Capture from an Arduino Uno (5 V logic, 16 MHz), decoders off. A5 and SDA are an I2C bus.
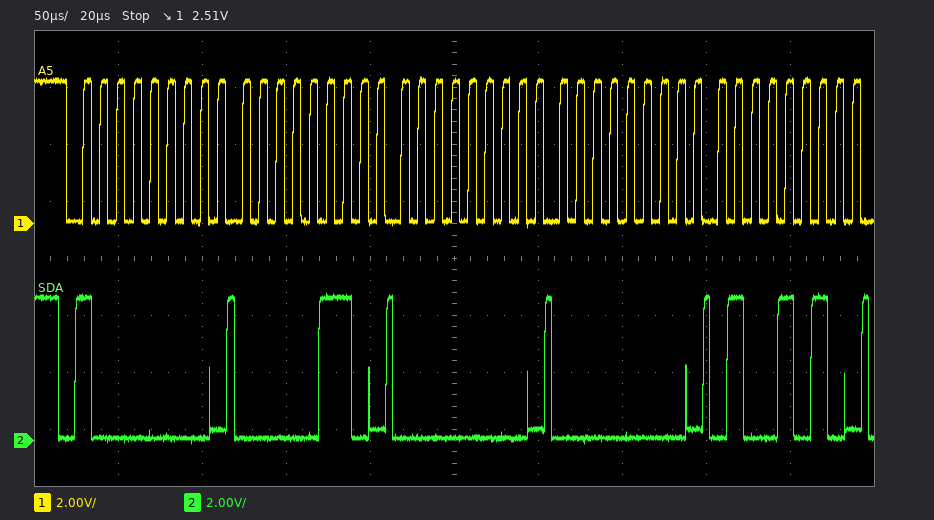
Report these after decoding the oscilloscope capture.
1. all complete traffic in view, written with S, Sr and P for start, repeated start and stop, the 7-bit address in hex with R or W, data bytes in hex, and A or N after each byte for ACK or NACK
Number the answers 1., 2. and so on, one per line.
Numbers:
1. S 40W A 06 A 00 A 00 A 4A A
